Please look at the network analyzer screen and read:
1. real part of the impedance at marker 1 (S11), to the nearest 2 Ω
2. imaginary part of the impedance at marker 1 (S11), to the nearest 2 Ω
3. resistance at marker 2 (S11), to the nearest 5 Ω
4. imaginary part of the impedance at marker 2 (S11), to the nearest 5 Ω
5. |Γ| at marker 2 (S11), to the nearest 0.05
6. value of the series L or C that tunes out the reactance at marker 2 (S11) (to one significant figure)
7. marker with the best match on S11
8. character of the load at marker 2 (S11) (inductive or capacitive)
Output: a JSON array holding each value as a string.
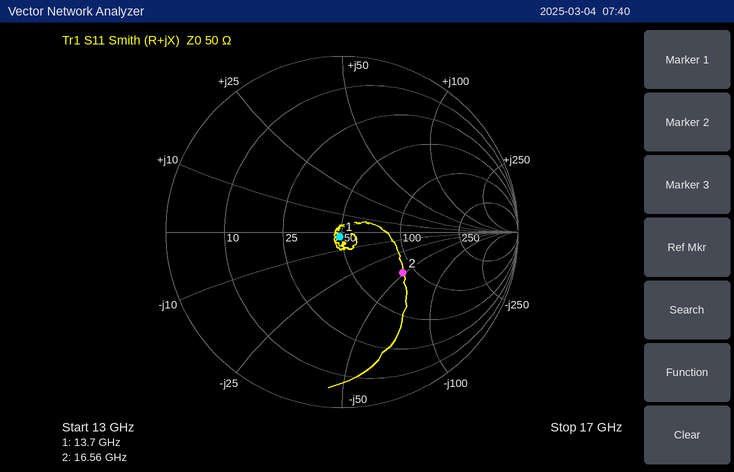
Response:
["48 Ω", "-2 Ω", "85 Ω", "-50 Ω", "0.40", "500 pH", "marker 1", "capacitive"]
